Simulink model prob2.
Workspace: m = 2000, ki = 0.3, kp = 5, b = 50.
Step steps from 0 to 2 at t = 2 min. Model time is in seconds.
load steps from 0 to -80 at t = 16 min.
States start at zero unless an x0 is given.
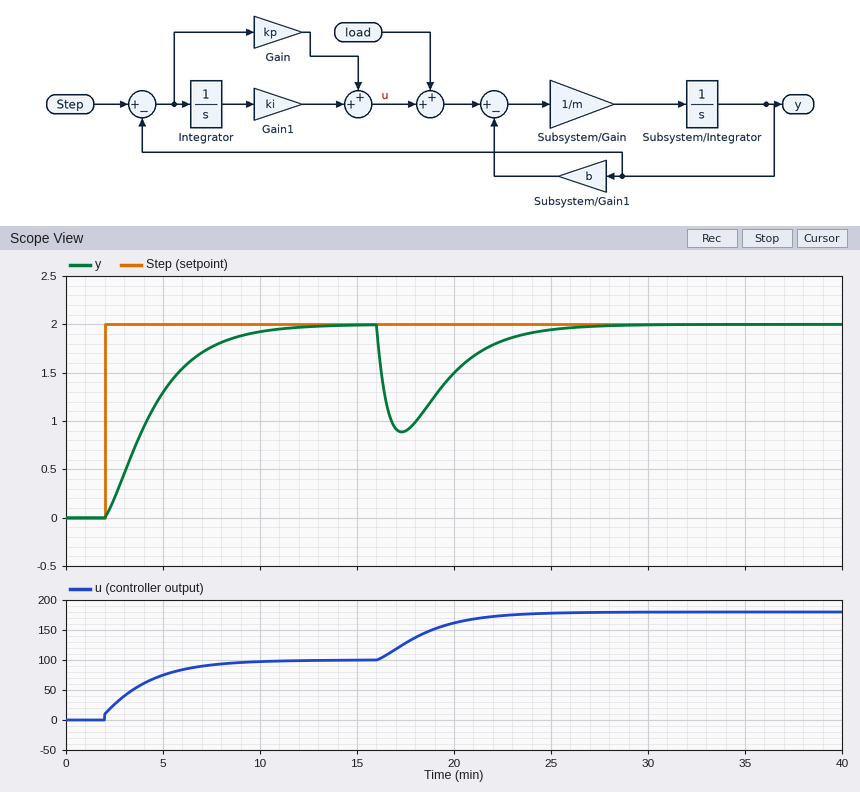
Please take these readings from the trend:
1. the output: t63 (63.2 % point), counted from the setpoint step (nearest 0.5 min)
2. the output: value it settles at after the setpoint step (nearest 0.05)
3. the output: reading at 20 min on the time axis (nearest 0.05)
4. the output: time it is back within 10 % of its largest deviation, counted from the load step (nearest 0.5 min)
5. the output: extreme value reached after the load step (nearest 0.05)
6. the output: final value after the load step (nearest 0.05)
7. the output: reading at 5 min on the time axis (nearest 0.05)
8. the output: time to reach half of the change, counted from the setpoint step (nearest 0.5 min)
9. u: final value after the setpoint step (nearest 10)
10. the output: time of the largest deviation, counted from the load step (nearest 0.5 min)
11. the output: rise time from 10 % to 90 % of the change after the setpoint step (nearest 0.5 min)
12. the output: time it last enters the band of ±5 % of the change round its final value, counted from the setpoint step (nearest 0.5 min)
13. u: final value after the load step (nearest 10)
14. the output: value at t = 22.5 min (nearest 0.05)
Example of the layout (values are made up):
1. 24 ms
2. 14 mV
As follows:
1. 3.0 min
2. 2.00
3. 1.50
4. 7.5 min
5. 0.90
6. 2.00
7. 1.30
8. 2.0 min
9. 100
10. 1.5 min
11. 5.5 min
12. 7.5 min
13. 180
14. 1.85
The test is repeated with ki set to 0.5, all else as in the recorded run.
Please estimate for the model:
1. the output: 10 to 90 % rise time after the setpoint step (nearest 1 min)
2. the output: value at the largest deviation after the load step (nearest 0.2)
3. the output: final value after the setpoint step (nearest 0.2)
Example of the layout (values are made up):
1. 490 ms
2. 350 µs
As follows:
1. 3 min
2. 1.0
3. 2.0
